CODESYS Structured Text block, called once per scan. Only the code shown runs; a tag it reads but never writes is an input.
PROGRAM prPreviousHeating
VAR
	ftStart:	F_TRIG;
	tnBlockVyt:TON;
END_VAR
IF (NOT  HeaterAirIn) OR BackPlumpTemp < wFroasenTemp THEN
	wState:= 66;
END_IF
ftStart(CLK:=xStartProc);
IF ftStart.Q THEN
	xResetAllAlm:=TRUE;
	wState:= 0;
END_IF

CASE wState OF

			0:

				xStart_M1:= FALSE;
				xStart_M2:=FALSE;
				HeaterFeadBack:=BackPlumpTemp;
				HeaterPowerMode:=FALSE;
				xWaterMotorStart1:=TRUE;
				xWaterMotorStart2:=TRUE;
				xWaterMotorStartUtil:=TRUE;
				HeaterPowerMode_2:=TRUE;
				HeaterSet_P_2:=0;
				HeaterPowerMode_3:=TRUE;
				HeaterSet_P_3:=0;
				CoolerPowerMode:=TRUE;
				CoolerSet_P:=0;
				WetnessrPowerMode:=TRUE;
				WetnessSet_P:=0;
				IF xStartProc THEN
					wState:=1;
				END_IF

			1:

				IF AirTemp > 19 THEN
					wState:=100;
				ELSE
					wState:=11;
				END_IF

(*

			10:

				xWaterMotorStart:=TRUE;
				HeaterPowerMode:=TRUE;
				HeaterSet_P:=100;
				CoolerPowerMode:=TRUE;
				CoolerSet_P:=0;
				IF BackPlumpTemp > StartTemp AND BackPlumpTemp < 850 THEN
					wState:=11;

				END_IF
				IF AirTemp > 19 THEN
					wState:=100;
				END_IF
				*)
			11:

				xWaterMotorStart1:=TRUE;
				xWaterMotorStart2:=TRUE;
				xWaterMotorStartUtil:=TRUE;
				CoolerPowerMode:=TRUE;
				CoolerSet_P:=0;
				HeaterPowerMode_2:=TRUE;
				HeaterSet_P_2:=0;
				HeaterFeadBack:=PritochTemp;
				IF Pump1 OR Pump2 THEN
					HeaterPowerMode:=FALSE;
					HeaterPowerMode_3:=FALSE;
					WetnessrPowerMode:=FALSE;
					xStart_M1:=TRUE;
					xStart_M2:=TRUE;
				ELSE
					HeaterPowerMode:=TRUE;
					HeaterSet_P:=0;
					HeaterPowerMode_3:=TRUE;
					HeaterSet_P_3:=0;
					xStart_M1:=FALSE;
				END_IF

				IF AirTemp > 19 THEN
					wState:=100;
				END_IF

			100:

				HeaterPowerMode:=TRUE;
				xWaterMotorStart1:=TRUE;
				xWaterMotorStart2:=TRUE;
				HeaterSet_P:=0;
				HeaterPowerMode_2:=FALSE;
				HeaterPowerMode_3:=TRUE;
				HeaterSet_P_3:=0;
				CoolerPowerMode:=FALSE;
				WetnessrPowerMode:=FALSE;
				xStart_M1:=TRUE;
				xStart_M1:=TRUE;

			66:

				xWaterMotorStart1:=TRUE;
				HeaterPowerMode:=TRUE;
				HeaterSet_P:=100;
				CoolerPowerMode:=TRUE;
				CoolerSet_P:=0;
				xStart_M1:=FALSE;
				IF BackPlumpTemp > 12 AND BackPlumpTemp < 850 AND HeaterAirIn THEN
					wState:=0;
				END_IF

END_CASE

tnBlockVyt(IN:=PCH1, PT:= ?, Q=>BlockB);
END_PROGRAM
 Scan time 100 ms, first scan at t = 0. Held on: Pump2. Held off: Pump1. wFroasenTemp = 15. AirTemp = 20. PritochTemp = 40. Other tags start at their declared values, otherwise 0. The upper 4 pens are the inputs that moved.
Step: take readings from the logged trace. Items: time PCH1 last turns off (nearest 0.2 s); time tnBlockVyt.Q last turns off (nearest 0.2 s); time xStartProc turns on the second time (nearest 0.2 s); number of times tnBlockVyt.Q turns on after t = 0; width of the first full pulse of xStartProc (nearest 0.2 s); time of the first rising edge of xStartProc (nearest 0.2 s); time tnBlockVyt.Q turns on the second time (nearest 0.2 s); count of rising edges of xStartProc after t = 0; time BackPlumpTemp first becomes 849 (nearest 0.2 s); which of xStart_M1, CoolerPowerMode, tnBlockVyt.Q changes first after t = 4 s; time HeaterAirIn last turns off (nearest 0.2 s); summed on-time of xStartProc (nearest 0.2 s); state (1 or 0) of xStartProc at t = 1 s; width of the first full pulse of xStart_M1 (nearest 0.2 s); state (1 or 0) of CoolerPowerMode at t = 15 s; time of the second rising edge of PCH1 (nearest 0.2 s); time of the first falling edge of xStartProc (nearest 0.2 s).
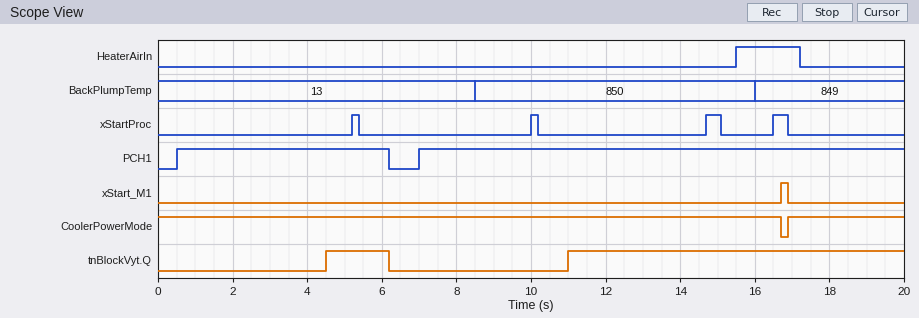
6.2 s
6.2 s
10.0 s
2
0.2 s
5.2 s
11.0 s
4
16.0 s
tnBlockVyt.Q
17.2 s
1.2 s
0
0.2 s
1
7.0 s
5.4 s
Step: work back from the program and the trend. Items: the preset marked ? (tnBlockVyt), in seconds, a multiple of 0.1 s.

4.0 s
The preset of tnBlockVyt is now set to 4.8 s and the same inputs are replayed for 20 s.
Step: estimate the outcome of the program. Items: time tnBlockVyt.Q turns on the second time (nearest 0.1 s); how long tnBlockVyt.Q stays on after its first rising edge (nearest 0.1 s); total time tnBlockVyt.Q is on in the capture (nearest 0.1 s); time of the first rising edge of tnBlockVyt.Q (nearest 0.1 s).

11.8 s
0.9 s
9.1 s
5.3 s
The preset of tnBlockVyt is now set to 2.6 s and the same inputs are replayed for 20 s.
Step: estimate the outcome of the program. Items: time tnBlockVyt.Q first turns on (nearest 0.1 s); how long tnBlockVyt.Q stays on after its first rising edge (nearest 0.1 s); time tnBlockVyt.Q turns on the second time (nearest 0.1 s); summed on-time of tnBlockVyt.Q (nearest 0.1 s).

3.1 s
3.1 s
9.6 s
13.5 s
